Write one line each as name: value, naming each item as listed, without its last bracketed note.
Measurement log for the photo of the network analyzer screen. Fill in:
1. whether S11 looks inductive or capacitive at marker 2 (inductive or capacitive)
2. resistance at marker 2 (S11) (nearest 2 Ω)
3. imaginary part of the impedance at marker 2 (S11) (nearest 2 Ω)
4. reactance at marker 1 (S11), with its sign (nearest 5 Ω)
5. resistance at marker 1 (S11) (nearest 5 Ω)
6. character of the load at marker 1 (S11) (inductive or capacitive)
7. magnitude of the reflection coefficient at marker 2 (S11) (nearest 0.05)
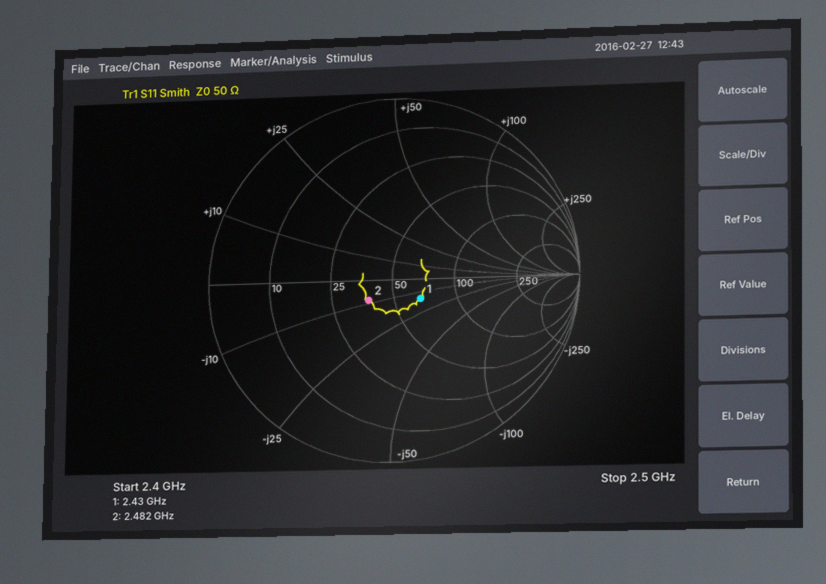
whether S11 looks inductive or capacitive at marker 2: capacitive
resistance at marker 2 (S11): 38 Ω
imaginary part of the impedance at marker 2 (S11): -8 Ω
reactance at marker 1 (S11), with its sign: -15 Ω
resistance at marker 1 (S11): 65 Ω
character of the load at marker 1 (S11): capacitive
magnitude of the reflection coefficient at marker 2 (S11): 0.15
